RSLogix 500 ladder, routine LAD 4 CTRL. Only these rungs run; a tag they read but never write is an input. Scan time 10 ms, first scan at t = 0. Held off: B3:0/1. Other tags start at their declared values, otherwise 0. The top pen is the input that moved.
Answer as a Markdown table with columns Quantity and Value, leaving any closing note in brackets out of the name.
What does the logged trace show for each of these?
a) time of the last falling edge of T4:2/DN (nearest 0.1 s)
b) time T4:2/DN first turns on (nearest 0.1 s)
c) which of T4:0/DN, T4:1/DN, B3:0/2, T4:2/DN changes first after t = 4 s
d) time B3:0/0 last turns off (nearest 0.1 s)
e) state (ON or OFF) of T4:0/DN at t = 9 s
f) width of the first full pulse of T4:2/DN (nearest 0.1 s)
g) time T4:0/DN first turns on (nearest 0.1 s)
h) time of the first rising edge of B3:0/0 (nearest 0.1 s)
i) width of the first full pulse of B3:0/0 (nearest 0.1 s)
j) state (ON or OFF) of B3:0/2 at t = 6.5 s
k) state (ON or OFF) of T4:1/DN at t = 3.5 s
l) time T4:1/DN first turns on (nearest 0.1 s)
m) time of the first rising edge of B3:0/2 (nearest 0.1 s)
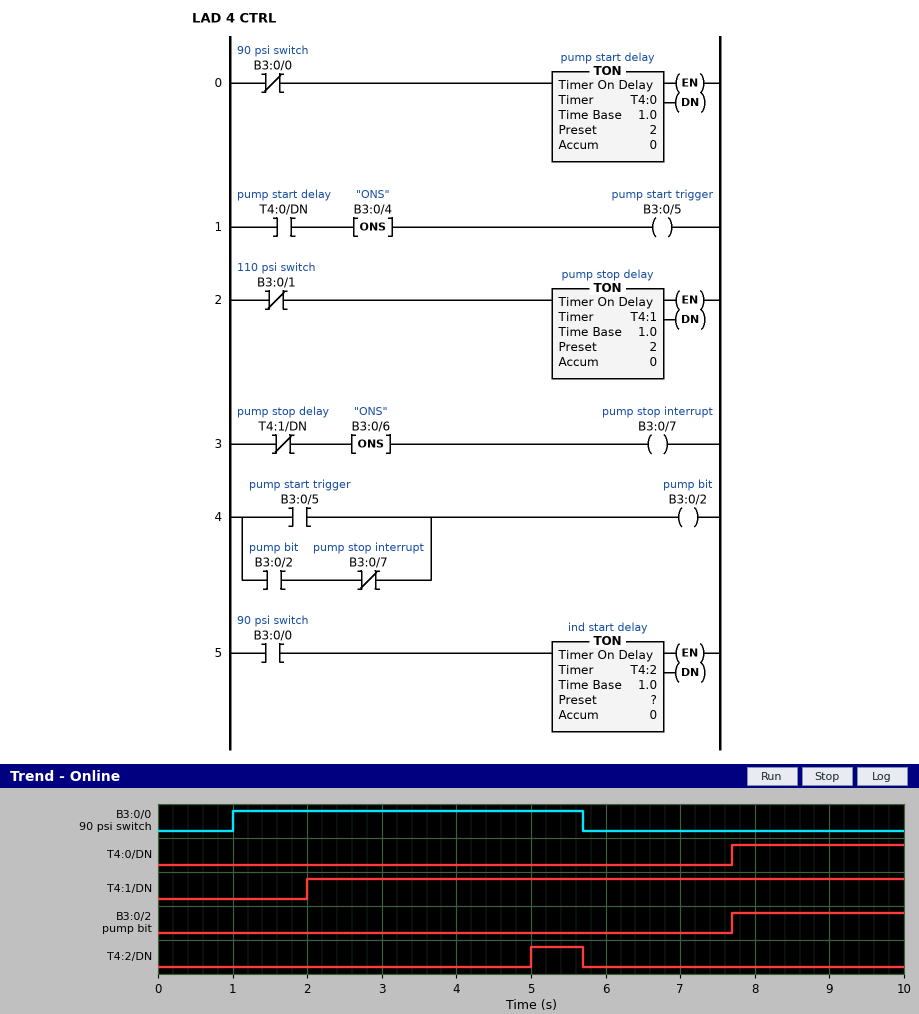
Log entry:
| Quantity | Value |
|---|---|
| time of the last falling edge of T4:2/DN | 5.7 s |
| time T4:2/DN first turns on | 5.0 s |
| which of T4:0/DN, T4:1/DN, B3:0/2, T4:2/DN changes first after t = 4 s | T4:2/DN |
| time B3:0/0 last turns off | 5.7 s |
| state (ON or OFF) of T4:0/DN at t = 9 s | ON |
| width of the first full pulse of T4:2/DN | 0.7 s |
| time T4:0/DN first turns on | 7.7 s |
| time of the first rising edge of B3:0/0 | 1.0 s |
| width of the first full pulse of B3:0/0 | 4.7 s |
| state (ON or OFF) of B3:0/2 at t = 6.5 s | OFF |
| state (ON or OFF) of T4:1/DN at t = 3.5 s | ON |
| time T4:1/DN first turns on | 2.0 s |
| time of the first rising edge of B3:0/2 | 7.7 s |
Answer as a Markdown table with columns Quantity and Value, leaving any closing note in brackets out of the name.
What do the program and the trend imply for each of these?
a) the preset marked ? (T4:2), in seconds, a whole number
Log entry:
| Quantity | Value |
|---|---|
| the preset marked ? (T4:2), in seconds, a whole number | 4 s |
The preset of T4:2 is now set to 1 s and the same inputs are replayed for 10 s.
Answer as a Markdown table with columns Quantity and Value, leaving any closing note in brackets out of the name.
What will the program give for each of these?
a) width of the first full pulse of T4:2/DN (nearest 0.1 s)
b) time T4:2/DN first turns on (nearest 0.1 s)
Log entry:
| Quantity | Value |
|---|---|
| width of the first full pulse of T4:2/DN | 3.7 s |
| time T4:2/DN first turns on | 2.0 s |
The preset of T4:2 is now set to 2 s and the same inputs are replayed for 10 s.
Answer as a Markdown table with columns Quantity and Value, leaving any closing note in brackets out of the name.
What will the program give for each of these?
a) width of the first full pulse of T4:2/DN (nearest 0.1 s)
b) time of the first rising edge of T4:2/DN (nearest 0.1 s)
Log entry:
| Quantity | Value |
|---|---|
| width of the first full pulse of T4:2/DN | 2.7 s |
| time of the first rising edge of T4:2/DN | 3.0 s |
